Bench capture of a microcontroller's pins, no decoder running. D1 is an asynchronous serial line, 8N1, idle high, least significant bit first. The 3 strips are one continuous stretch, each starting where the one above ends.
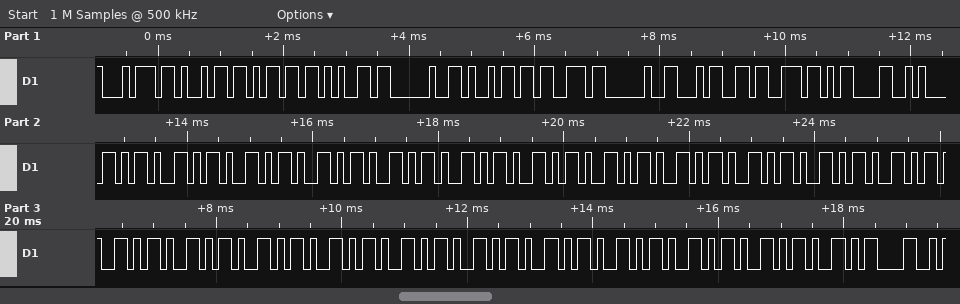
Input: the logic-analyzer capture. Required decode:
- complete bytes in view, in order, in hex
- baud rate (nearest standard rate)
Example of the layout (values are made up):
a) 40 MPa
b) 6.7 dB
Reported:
a) 74 69 6D 65 20 69 73 20 34 73 0D 0A 2D 2D 2D 2D 2D 2D 2D 2D 2D 2D 2D 2D 2D 2D 2D 2D 2D 2D 2D 2D 2D 2D 0D
b) 9600 baud
